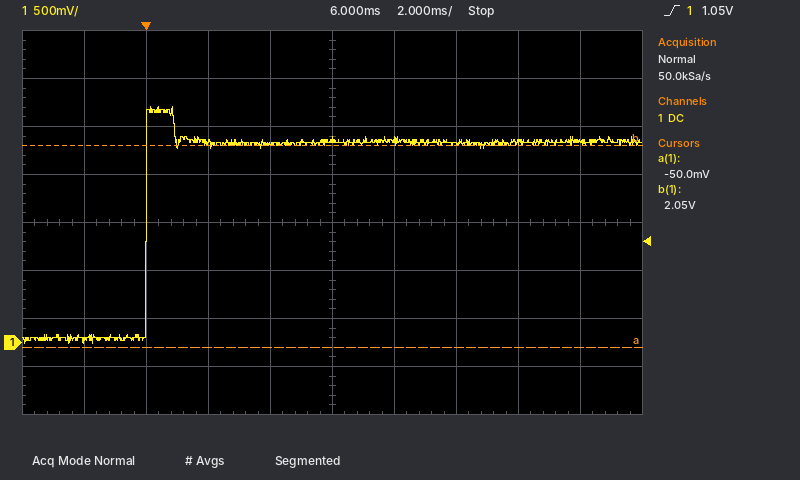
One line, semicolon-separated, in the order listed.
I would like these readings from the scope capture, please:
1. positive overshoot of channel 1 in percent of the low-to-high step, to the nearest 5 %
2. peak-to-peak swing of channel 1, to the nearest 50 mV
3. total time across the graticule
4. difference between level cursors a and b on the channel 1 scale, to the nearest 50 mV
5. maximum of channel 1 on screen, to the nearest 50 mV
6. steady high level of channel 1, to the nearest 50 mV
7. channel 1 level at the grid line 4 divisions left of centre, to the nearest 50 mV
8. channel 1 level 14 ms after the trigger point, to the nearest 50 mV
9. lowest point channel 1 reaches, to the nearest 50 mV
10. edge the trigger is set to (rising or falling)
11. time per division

20 %; 2.45 V; 20 ms; 2.10 V; 2.45 V; 2.10 V; 0 mV; 2.10 V; 0 mV; rising; 2 ms
